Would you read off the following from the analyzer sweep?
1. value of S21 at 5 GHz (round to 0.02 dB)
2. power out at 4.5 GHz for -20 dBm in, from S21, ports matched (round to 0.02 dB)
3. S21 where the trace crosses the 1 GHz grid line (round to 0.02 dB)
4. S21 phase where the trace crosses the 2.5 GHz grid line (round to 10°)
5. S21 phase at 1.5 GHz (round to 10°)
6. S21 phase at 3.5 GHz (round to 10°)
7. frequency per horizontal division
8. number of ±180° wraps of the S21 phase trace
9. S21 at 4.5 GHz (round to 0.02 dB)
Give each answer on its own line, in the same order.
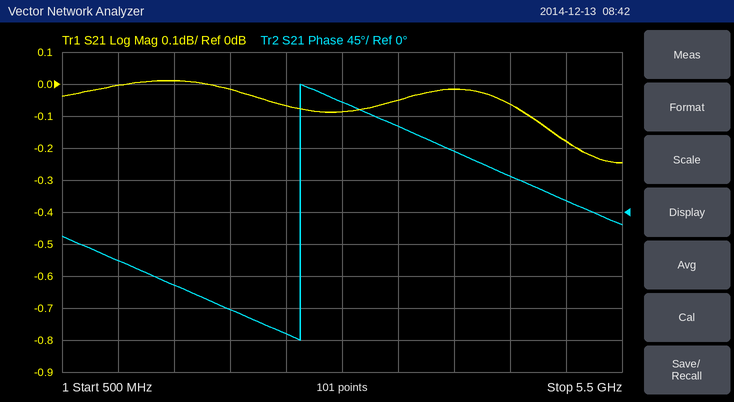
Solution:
-0.18 dB
-20.06 dBm
0.00 dB
-170°
-100°
120°
500 MHz
1
-0.06 dB
